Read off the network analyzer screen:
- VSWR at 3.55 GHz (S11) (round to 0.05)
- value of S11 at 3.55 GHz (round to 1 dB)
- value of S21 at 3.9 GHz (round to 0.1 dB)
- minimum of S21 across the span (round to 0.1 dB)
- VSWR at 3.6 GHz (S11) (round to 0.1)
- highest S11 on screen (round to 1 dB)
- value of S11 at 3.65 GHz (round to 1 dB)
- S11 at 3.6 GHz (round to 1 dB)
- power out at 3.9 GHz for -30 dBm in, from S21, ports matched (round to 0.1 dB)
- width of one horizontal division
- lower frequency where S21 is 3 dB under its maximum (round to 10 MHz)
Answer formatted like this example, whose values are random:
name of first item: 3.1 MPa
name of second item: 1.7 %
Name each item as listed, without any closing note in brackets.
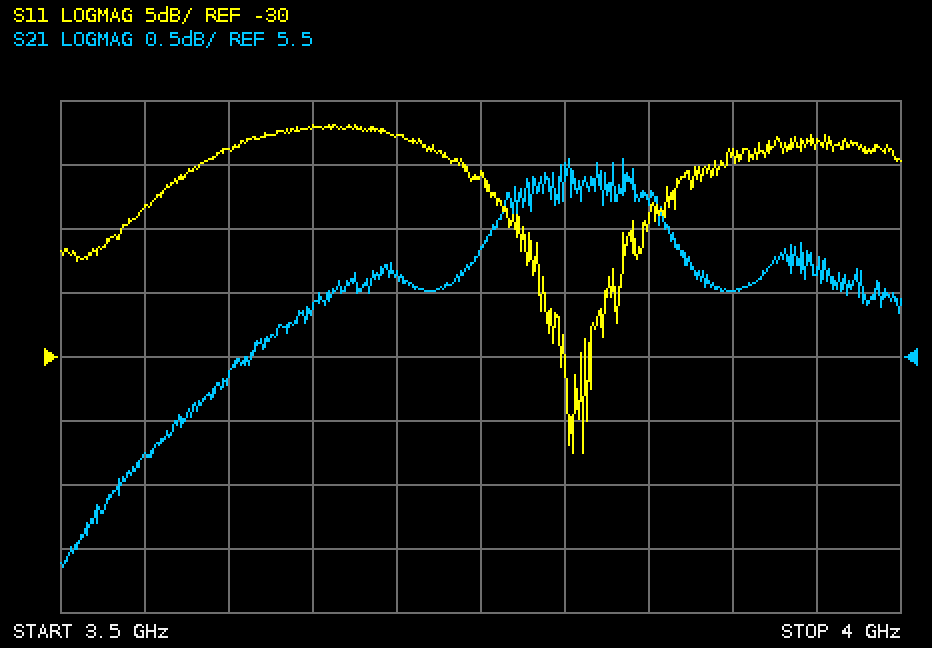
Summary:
VSWR at 3.55 GHz (S11): 1.30
value of S11 at 3.55 GHz: -18 dB
value of S21 at 3.9 GHz: 6.0 dB
minimum of S21 across the span: 3.9 dB
VSWR at 3.6 GHz (S11): 1.5
highest S11 on screen: -12 dB
value of S11 at 3.65 GHz: -12 dB
S11 at 3.6 GHz: -14 dB
power out at 3.9 GHz for -30 dBm in, from S21, ports matched: -24.0 dBm
width of one horizontal division: 50 MHz
lower frequency where S21 is 3 dB under its maximum: 3.51 GHz
